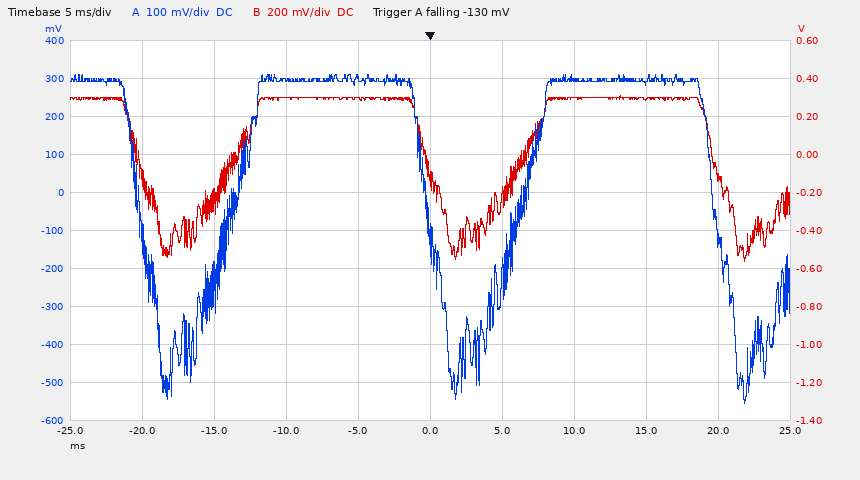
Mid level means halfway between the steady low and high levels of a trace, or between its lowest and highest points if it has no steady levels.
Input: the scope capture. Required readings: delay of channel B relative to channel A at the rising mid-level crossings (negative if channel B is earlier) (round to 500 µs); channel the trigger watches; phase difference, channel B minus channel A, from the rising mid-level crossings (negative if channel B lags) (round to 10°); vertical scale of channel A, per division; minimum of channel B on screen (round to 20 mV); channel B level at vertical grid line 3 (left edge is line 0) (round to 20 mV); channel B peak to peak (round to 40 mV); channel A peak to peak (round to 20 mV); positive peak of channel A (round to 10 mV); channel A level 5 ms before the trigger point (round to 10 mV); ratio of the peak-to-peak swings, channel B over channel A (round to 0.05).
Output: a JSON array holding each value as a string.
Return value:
["0.0 ms", "channel A", "0°", "100 mV", "-560 mV", "300 mV", "880 mV", "860 mV", "310 mV", "300 mV", "1.00"]
